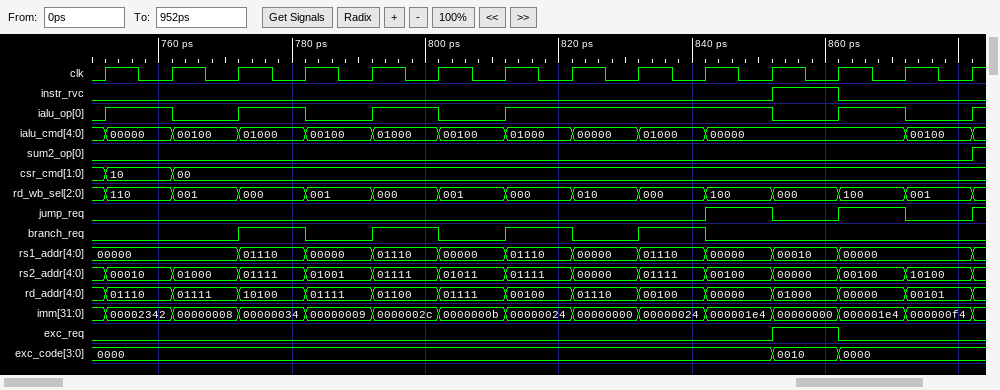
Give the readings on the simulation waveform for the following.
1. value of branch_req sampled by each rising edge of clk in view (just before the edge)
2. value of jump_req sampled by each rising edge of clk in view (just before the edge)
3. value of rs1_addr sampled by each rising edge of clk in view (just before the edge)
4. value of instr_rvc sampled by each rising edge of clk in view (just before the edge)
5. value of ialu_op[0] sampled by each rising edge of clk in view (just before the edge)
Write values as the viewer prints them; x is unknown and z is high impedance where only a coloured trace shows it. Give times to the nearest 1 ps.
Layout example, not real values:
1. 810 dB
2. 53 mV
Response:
1. 0 0 0 1 0 1 0 1 0 1 0 0 0 0
2. 0 0 0 0 0 0 0 0 0 0 1 0 1 0
3. 00000, 00000, 00000, 01110, 00000, 01110, 00000, 01110, 00000, 01110, 00000, 00010, 00000, 00000
4. 0 0 0 0 0 0 0 0 0 0 0 1 0 0
5. 0 1 0 1 0 1 0 1 1 1 1 0 1 0
